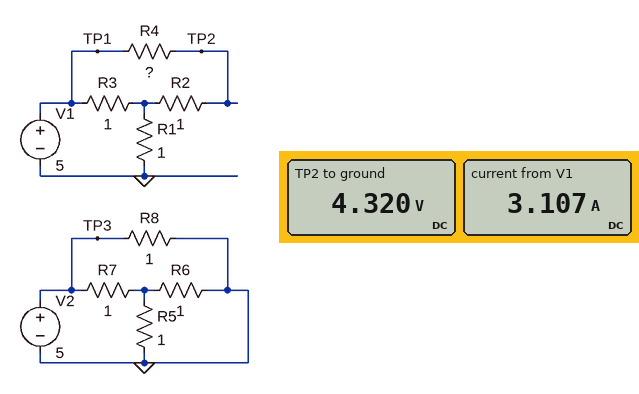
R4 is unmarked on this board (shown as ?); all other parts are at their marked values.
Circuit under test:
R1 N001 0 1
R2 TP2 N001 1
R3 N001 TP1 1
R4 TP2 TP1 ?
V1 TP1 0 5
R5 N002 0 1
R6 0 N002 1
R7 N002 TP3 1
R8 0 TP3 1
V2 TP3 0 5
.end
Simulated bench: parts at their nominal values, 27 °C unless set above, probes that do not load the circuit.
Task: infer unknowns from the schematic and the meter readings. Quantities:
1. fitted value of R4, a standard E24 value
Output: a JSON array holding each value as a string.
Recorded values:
["0.56 Ω"]
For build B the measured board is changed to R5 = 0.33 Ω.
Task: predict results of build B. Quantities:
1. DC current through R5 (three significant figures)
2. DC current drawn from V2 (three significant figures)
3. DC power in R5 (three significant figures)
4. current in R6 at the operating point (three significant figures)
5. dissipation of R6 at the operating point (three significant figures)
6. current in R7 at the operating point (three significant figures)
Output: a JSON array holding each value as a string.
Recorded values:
["3.01 A", "9.01 A", "2.99 W", "994 mA", "988 mW", "4.01 A"]
